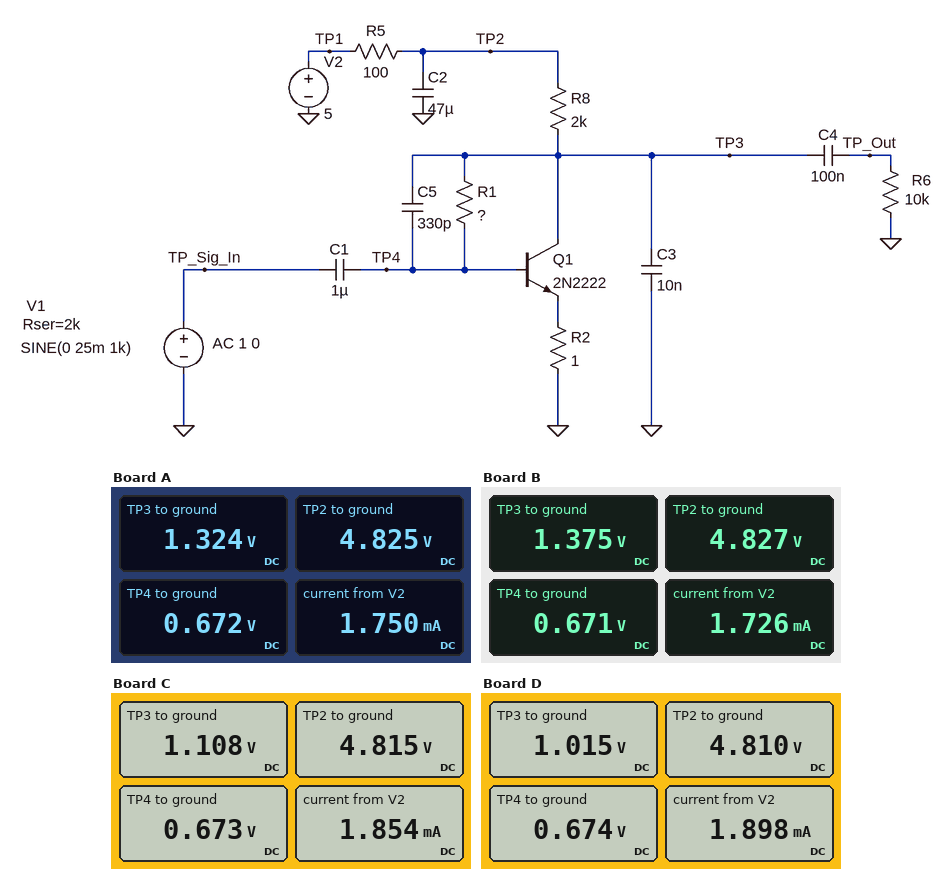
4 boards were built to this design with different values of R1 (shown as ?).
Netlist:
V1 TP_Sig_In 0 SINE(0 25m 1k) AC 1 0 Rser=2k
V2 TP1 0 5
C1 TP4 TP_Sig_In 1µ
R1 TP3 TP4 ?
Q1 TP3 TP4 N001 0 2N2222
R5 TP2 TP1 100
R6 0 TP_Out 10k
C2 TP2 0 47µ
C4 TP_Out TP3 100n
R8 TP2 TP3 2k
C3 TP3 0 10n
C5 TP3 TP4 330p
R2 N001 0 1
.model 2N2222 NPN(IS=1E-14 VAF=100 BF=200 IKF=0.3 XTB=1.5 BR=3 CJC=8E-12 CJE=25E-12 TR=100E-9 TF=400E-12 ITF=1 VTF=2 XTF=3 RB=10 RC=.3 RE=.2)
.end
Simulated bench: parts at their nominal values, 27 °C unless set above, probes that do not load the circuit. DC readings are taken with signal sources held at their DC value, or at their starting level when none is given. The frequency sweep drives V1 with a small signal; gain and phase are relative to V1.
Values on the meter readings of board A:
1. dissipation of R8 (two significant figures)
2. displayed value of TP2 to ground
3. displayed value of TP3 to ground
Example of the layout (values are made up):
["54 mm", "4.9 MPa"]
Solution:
["6.1 mW", "4.825 V", "1.324 V"]
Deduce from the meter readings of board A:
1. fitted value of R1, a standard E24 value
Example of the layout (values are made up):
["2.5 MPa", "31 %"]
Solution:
["75 kΩ"]
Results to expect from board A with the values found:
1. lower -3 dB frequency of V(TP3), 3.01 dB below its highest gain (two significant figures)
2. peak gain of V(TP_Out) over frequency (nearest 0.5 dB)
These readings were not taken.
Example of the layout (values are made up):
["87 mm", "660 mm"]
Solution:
["55 Hz", "27.0 dB"]
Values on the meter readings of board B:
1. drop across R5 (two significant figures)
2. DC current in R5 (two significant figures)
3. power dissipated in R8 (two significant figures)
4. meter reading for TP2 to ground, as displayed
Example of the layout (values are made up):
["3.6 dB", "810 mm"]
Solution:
["170 mV", "1.7 mA", "6.0 mW", "4.827 V"]
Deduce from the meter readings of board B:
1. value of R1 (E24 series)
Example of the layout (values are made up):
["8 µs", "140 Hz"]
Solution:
["82 kΩ"]
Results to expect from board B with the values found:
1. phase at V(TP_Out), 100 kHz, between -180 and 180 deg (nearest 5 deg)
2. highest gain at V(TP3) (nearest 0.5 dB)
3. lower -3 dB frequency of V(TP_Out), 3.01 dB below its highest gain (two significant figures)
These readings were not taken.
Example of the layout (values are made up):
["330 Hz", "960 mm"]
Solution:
["90 deg", "27.5 dB", "160 Hz"]
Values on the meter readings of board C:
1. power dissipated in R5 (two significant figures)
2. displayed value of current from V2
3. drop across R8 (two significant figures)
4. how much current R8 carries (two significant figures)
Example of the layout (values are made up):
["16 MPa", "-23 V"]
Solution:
["340 µW", "1.854 mA", "3.7 V", "1.9 mA"]
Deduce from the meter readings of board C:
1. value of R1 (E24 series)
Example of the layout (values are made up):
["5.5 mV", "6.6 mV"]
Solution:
["47 kΩ"]
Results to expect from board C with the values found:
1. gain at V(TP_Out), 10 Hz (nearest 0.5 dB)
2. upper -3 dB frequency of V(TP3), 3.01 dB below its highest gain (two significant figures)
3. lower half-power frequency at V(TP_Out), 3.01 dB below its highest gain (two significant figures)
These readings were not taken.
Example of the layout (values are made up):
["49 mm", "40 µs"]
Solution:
["-16.0 dB", "10 kHz", "170 Hz"]
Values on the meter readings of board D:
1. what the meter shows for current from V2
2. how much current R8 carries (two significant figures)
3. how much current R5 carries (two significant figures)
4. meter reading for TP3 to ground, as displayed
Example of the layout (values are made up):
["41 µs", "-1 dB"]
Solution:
["1.898 mA", "1.9 mA", "1.9 mA", "1.015 V"]
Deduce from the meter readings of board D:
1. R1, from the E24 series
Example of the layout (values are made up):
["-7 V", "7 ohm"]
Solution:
["36 kΩ"]
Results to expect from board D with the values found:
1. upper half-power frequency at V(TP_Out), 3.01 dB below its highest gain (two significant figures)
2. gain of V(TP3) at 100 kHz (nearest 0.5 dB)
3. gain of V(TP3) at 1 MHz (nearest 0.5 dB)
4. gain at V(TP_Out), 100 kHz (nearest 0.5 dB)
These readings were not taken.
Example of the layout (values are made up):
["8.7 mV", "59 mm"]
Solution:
["13 kHz", "4.5 dB", "-17.5 dB", "4.5 dB"]
